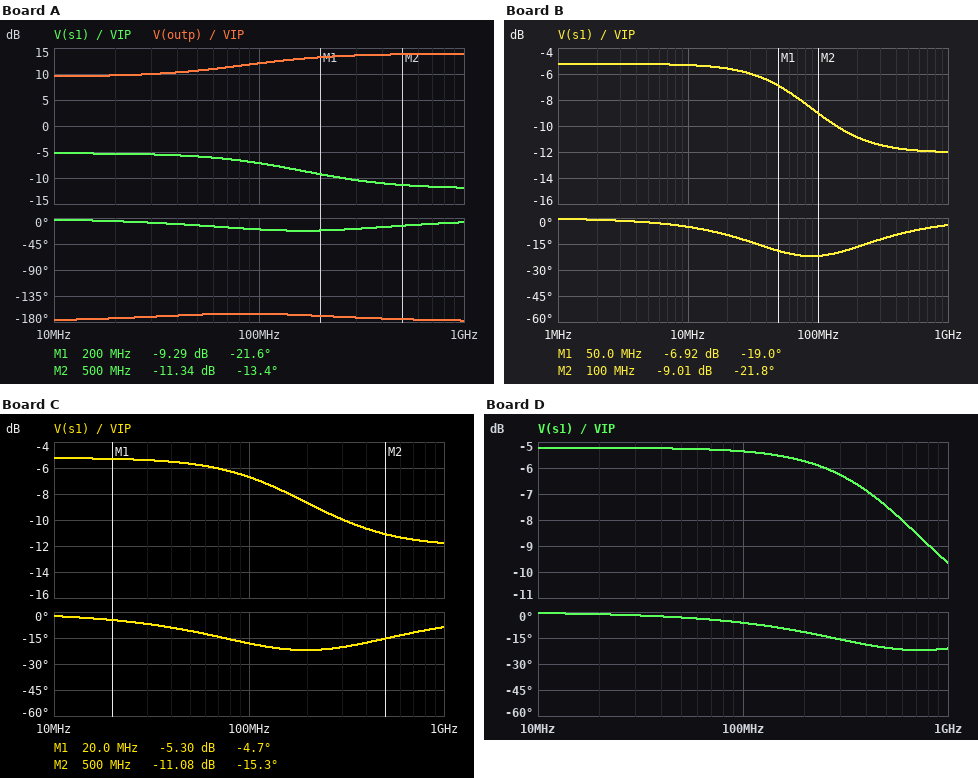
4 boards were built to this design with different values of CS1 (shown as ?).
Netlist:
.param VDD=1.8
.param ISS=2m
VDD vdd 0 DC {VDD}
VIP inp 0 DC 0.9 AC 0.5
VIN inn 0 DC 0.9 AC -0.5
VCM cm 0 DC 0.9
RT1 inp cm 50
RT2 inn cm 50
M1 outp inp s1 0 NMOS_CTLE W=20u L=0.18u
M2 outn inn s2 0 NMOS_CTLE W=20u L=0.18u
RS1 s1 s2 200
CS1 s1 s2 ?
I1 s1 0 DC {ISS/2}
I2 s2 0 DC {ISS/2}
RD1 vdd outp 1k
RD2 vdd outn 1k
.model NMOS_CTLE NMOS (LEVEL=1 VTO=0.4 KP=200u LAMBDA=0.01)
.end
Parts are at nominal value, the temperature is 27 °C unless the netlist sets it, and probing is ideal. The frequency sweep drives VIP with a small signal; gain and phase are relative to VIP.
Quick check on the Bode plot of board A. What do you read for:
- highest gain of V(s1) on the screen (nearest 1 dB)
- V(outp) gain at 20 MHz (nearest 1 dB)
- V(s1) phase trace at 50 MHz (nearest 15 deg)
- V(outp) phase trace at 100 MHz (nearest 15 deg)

-5 dB
10 dB
-15 deg
-165 deg
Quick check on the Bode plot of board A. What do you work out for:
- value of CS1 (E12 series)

12 pF
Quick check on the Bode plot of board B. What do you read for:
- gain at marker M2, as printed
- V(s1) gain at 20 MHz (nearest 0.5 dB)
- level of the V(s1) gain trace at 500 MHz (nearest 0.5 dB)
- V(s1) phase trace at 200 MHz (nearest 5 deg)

-9.01 dB
-5.5 dB
-12.0 dB
-15 deg
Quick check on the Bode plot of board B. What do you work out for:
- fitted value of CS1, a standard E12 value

22 pF
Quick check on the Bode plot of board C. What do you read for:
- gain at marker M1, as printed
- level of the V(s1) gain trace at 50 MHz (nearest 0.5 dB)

-5.30 dB
-5.5 dB
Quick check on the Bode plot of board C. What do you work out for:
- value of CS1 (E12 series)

10 pF
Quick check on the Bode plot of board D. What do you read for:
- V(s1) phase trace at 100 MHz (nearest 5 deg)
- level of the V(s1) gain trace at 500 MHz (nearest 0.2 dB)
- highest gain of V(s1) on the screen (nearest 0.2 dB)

-5 deg
-7.4 dB
-5.2 dB
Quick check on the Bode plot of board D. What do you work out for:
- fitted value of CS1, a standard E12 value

2.7 pF
